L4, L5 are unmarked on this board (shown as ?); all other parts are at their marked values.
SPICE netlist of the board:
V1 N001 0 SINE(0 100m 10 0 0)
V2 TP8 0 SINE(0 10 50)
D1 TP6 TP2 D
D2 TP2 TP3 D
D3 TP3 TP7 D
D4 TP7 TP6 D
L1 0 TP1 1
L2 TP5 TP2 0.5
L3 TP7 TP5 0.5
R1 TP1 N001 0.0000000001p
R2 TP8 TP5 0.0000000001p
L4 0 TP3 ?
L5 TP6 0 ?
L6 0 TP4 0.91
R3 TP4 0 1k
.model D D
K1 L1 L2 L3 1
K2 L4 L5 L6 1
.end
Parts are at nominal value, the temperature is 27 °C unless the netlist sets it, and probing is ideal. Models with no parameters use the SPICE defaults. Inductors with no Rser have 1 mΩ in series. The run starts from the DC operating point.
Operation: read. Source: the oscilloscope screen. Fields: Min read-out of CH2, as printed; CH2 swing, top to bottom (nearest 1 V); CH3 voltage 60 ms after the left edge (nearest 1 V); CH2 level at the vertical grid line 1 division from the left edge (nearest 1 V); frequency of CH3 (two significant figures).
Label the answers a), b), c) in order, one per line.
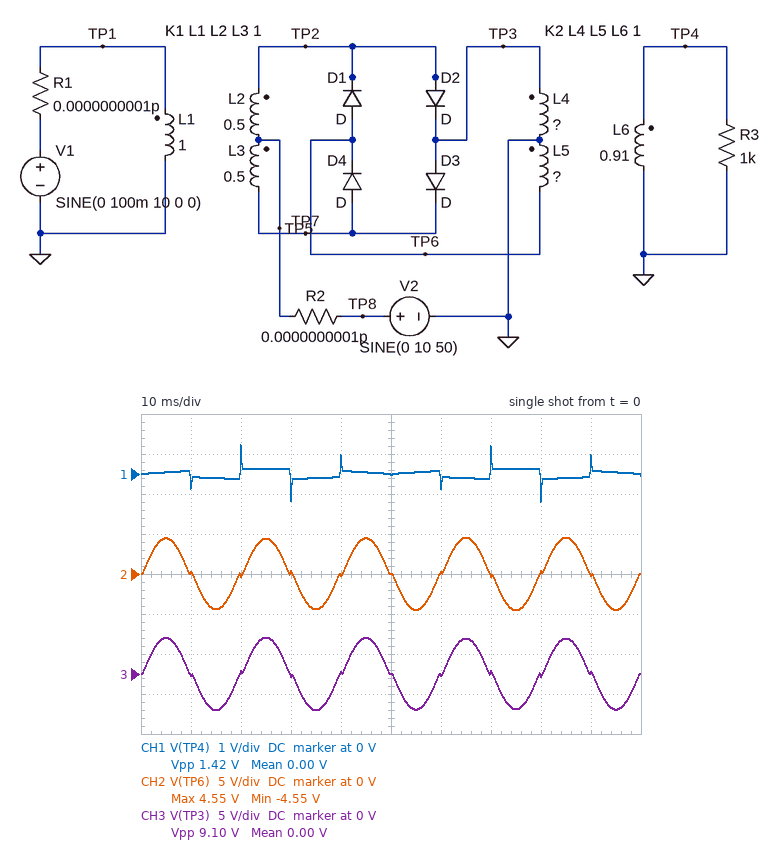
a) -4.55 V
b) 9 V
c) 0 V
d) 0 V
e) 50 Hz
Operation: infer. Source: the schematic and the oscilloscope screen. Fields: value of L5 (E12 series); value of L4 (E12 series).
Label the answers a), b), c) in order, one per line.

a) 270 mH
b) 270 mH
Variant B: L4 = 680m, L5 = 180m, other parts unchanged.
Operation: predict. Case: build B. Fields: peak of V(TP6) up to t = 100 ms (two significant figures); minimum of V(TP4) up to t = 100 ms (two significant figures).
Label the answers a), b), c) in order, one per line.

a) 3.8 V
b) -3.6 V
